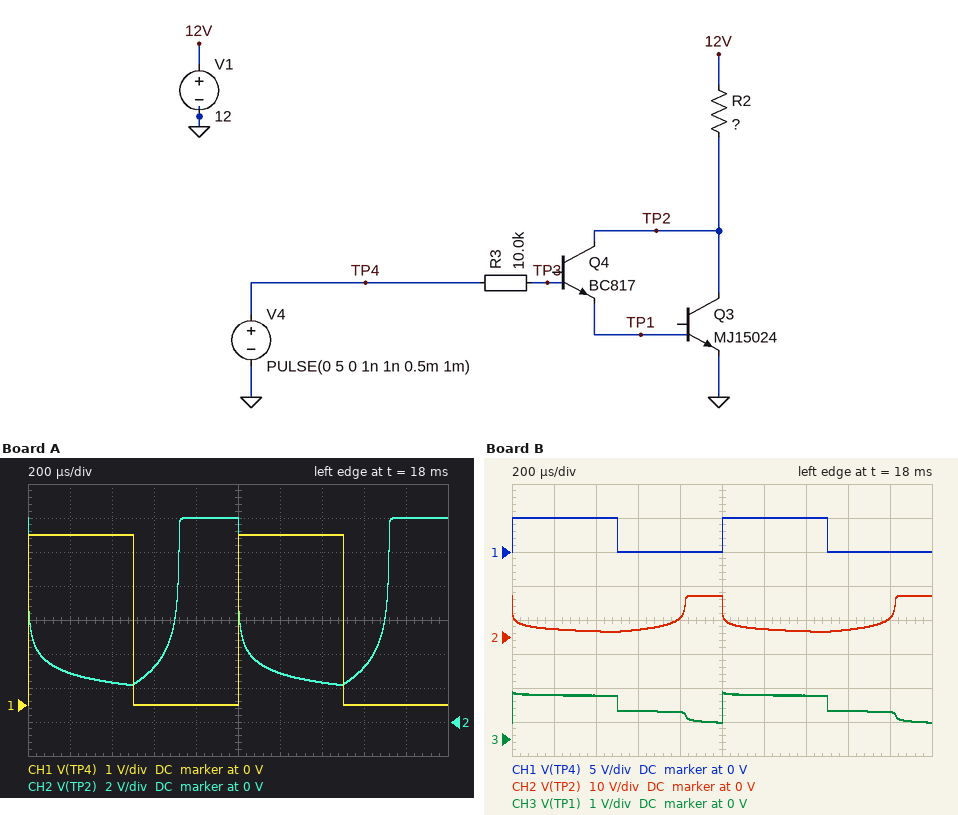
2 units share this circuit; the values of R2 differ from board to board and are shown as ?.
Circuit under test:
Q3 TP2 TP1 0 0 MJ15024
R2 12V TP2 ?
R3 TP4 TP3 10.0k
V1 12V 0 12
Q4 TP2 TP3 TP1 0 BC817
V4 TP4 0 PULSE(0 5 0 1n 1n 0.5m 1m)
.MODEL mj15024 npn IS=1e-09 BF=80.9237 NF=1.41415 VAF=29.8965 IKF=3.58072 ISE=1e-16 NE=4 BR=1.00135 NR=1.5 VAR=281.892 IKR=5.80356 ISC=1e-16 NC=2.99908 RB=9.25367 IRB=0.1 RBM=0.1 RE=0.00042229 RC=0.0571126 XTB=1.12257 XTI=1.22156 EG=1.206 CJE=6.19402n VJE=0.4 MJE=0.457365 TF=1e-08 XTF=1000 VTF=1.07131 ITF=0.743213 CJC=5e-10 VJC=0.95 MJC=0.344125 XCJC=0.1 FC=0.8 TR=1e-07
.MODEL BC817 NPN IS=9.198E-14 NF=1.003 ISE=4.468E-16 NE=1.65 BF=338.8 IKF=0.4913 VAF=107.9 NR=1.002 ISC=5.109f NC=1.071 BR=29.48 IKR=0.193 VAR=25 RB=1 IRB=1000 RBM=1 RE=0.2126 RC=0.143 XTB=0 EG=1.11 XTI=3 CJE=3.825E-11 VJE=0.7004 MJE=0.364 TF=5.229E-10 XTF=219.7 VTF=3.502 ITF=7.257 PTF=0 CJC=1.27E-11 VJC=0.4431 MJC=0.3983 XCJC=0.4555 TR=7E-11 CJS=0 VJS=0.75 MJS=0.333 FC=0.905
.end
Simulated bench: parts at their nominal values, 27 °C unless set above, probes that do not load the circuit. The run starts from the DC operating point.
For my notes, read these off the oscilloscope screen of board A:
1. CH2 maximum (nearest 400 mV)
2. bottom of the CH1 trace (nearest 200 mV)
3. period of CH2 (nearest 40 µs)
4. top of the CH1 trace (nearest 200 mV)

12.0 V
0 V
1.00 ms
5.0 V
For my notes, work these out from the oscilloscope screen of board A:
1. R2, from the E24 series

3 Ω
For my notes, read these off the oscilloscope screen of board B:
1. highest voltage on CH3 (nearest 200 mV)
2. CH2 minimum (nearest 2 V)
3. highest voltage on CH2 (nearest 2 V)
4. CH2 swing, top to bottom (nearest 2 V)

1.4 V
2 V
12 V
10 V
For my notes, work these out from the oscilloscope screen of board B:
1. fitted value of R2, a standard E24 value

3.6 Ω
